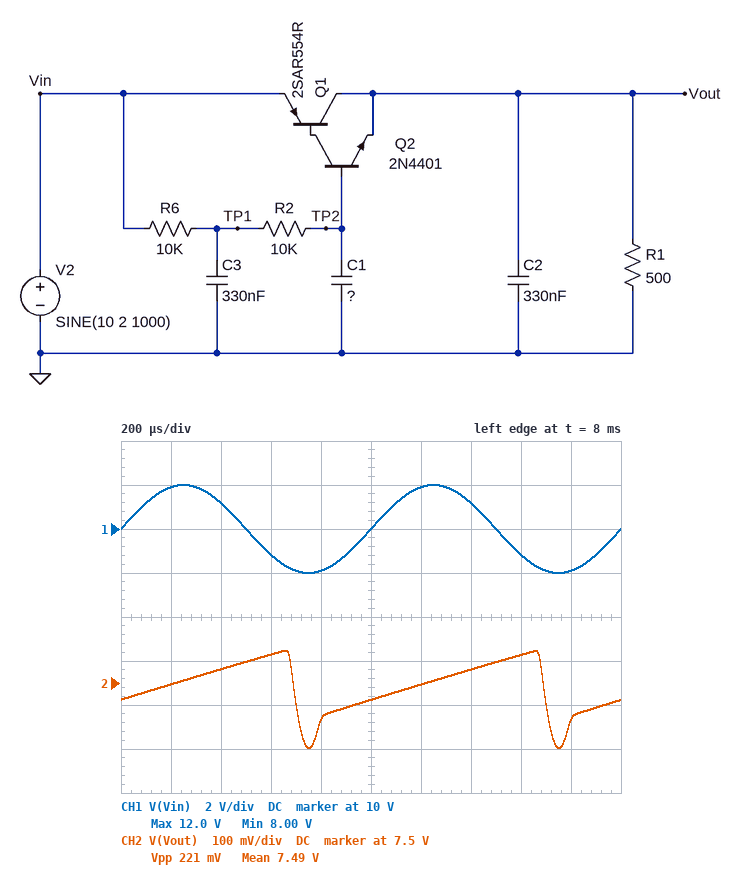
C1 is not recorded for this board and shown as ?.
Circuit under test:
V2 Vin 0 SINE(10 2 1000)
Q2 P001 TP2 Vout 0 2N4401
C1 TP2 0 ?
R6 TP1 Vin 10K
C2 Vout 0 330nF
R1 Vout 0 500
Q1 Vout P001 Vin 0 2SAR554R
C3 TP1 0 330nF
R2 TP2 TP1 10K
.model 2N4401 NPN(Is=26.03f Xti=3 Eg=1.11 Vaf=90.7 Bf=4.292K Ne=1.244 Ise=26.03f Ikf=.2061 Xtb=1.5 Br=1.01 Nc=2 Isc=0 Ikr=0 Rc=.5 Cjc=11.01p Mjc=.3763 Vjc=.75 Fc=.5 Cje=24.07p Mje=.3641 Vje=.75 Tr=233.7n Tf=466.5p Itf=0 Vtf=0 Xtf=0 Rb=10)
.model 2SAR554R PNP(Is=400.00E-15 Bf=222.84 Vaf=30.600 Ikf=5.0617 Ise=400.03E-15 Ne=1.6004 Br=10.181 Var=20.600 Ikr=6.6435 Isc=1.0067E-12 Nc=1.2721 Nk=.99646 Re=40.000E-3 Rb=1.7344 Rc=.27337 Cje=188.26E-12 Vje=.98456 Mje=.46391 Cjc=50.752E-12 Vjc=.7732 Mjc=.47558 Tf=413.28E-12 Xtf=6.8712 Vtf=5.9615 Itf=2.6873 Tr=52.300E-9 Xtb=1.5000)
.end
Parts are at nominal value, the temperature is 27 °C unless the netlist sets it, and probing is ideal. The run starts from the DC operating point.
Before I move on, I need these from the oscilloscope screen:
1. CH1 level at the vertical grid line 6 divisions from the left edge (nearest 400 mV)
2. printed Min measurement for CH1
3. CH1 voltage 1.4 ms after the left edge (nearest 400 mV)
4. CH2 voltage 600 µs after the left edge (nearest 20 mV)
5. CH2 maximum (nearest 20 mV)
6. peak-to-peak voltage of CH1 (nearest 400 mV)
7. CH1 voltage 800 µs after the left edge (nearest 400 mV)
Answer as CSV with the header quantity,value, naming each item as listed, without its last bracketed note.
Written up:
quantity,value
CH1 level at the vertical grid line 6 divisions from the left edge,12.0 V
printed Min measurement for CH1,8.00 V
CH1 voltage 1.4 ms after the left edge,11.2 V
CH2 voltage 600 µs after the left edge,7.56 V
CH2 maximum,7.58 V
peak-to-peak voltage of CH1,4.0 V
CH1 voltage 800 µs after the left edge,8.0 V
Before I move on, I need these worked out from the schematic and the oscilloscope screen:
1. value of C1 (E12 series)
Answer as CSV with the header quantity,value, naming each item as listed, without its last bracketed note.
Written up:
quantity,value
value of C1,560 nF
